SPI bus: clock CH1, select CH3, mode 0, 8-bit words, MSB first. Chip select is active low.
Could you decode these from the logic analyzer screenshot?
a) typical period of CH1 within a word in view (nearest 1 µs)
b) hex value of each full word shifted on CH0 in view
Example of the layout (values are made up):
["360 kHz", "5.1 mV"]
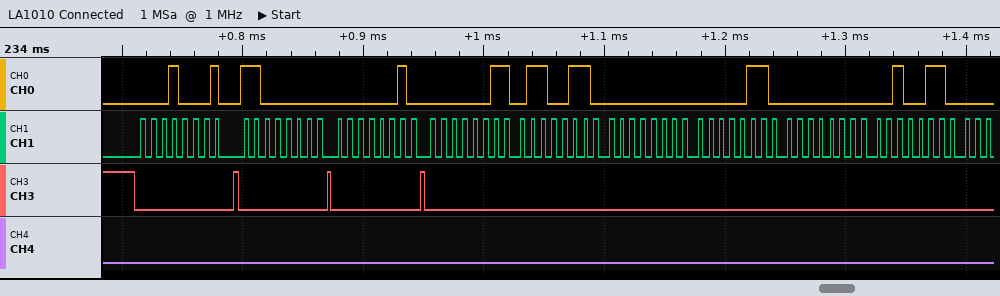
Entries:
["9 µs", "11, C0, 02, 03, 66, 00, 06, 00, 26"]
